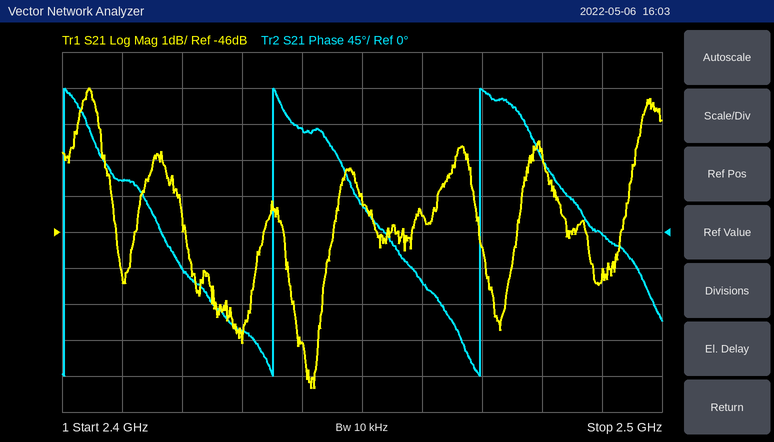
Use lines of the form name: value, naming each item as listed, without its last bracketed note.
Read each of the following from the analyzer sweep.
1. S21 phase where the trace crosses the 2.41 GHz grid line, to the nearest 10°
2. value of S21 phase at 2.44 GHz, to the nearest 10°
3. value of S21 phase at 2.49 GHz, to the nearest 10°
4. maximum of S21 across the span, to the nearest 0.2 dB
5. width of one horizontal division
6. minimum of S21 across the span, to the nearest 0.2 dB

S21 phase where the trace crosses the 2.41 GHz grid line, to the nearest 10°: 60°
value of S21 phase at 2.44 GHz, to the nearest 10°: 130°
value of S21 phase at 2.49 GHz, to the nearest 10°: 0°
maximum of S21 across the span, to the nearest 0.2 dB: -42.0 dB
width of one horizontal division: 10 MHz
minimum of S21 across the span, to the nearest 0.2 dB: -50.4 dB
